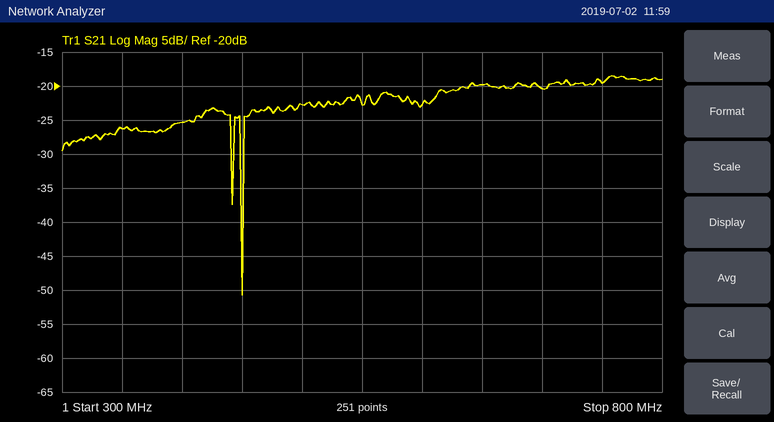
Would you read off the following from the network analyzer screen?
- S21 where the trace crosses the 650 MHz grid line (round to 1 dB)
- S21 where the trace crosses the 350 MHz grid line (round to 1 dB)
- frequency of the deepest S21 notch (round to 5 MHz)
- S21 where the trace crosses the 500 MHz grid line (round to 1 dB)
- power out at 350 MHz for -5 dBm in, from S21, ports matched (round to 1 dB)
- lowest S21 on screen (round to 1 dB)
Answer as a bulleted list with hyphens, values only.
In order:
- -20 dB
- -26 dB
- 450 MHz
- -23 dB
- -31 dBm
- -51 dB
